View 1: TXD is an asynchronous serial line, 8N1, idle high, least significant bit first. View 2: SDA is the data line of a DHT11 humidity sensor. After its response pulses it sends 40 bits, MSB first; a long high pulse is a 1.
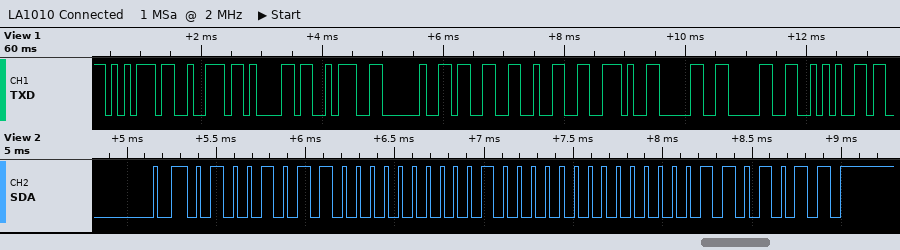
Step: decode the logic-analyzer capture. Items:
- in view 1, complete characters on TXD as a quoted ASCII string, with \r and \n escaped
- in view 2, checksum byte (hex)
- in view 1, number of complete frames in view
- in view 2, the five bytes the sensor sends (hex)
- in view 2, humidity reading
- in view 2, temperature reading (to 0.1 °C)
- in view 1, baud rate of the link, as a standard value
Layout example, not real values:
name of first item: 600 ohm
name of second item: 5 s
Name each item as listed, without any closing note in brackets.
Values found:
in view 1, complete characters on TXD as a quoted ASCII string, with \r and \n escaped: "ura: 32.00*"
in view 2, checksum byte: 0x6B
in view 1, number of complete frames in view: 11
in view 2, the five bytes the sensor sends: 4B 00 20 00 6B
in view 2, humidity reading: 75 %
in view 2, temperature reading: 32.0 °C
in view 1, baud rate of the link, as a standard value: 9600 baud
